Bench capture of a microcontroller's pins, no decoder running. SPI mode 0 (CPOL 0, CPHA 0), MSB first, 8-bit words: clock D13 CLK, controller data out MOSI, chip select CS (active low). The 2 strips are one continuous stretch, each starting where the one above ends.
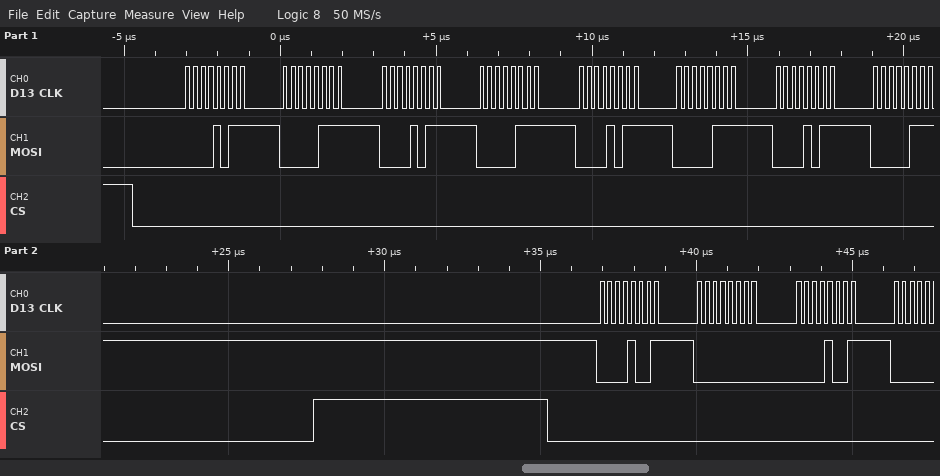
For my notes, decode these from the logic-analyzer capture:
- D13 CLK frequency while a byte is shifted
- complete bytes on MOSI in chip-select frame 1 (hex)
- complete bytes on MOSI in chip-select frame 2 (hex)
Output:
4 MHz
0B 07 0B 07 0B 07 0B 07
09 00 09
